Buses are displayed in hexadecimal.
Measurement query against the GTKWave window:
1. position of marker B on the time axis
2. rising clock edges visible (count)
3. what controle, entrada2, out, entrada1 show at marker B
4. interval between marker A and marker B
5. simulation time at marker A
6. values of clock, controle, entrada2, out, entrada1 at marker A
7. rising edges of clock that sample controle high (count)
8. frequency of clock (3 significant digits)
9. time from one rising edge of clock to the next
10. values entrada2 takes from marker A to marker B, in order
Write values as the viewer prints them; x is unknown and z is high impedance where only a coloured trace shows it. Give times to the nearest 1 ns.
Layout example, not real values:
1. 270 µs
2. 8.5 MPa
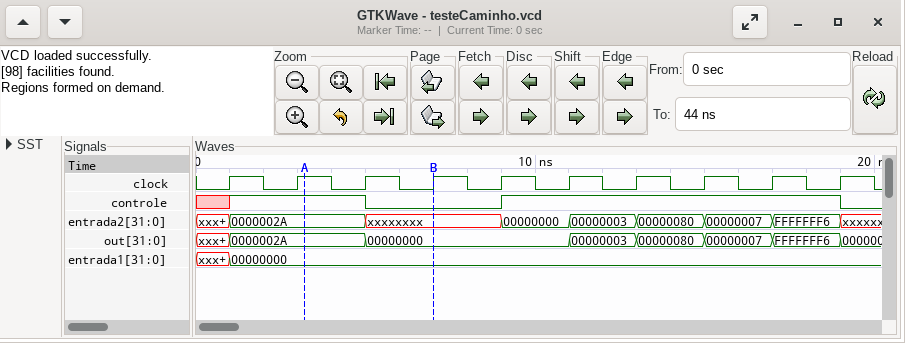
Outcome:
1. 7 ns
2. 10
3. controle=0, entrada2=xxxxxxxx, out=00000000, entrada1=00000000
4. 4 ns
5. 3 ns
6. clock=1, controle=1, entrada2=0000002A, out=0000002A, entrada1=00000000
7. 7
8. 500 MHz
9. 2 ns
10. 0000002A, xxxxxxxx
